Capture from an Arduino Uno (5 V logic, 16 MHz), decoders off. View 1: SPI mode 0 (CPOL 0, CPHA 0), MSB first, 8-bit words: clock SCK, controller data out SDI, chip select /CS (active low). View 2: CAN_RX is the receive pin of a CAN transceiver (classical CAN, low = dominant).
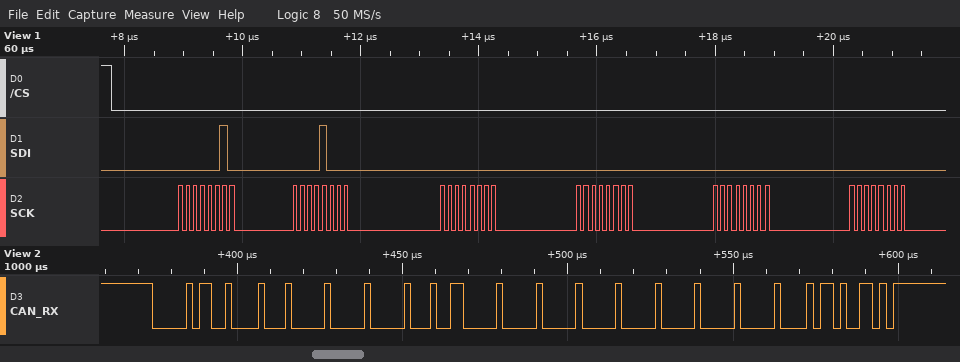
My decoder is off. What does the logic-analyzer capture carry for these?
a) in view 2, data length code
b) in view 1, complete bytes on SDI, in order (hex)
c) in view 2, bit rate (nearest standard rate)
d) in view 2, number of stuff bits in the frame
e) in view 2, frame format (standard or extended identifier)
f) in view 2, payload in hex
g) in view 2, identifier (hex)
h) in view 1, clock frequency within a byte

8
02 08 00 00 00 00
500 kbit/s
12
standard
80 00 13 00 00 00 00 00
0x032
8 MHz
